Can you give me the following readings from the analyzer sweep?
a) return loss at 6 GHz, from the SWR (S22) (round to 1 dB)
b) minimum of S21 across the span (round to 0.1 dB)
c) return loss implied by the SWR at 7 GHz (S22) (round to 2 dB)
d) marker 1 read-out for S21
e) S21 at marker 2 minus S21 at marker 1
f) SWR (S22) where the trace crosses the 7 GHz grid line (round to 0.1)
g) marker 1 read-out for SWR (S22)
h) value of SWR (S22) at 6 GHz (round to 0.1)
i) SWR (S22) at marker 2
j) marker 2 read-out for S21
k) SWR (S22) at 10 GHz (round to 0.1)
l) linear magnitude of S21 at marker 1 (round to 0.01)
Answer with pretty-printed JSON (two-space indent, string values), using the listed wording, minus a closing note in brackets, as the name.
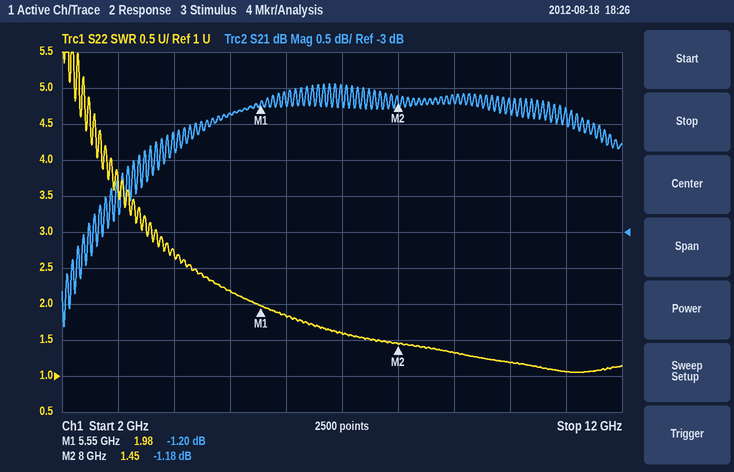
{
  "return loss at 6 GHz, from the SWR (S22)": "11 dB",
  "minimum of S21 across the span": "-4.3 dB",
  "return loss implied by the SWR at 7 GHz (S22)": "12 dB",
  "marker 1 read-out for S21": "-1.20 dB",
  "S21 at marker 2 minus S21 at marker 1": "0.02 dB",
  "SWR (S22) where the trace crosses the 7 GHz grid line": "1.6",
  "marker 1 read-out for SWR": "1.98",
  "value of SWR (S22) at 6 GHz": "1.8",
  "SWR (S22) at marker 2": "1.45",
  "marker 2 read-out for S21": "-1.18 dB",
  "SWR (S22) at 10 GHz": "1.2",
  "linear magnitude of S21 at marker 1": "0.87"
}
